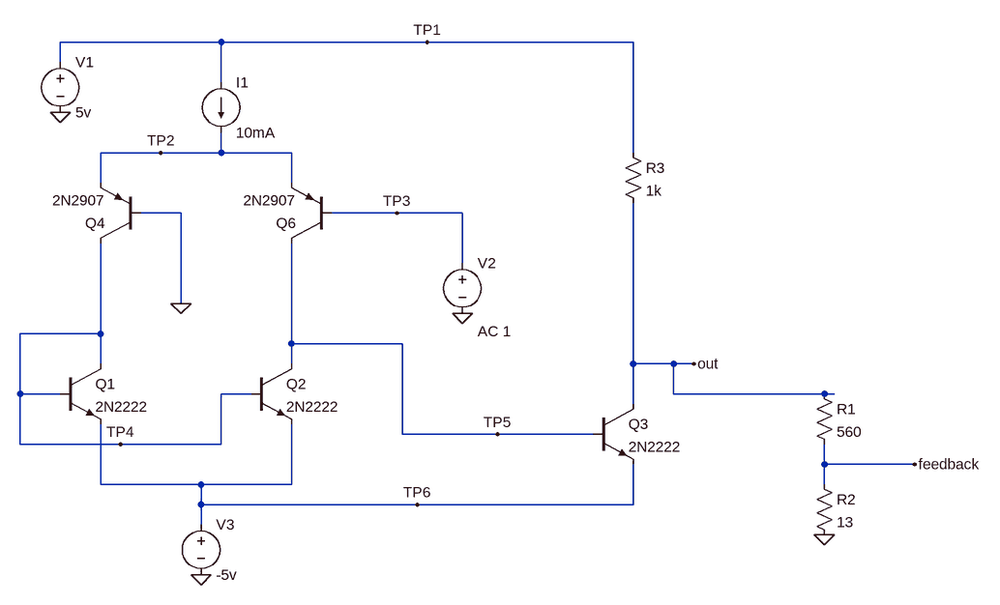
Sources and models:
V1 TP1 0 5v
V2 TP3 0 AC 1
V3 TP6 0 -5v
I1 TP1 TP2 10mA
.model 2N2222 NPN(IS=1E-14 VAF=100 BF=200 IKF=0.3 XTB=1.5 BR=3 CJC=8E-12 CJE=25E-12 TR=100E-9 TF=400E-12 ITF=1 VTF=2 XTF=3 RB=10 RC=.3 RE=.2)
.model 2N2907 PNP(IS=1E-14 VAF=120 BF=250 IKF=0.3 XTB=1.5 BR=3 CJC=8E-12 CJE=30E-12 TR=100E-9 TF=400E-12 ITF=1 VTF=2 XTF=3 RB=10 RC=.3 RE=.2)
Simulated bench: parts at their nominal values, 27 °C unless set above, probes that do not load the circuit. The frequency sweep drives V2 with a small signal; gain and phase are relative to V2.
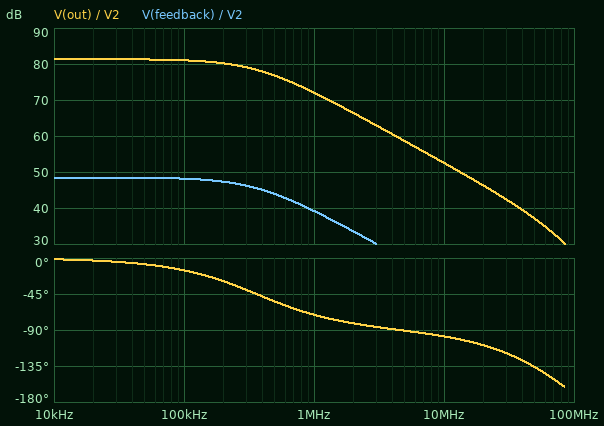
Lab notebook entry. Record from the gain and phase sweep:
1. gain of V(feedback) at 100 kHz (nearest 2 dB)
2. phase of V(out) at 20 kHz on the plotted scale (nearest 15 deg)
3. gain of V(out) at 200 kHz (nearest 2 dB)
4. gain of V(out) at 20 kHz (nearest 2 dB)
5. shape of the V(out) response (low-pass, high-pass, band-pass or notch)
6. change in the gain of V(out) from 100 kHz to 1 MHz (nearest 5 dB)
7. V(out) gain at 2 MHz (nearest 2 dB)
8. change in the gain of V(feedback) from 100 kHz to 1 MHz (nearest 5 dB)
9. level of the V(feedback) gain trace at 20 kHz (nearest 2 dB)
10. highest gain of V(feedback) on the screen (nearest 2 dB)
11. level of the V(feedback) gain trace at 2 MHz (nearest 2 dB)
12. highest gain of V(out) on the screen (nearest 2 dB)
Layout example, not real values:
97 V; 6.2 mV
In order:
48 dB; 0 deg; 80 dB; 82 dB; low-pass; -10 dB; 66 dB; -10 dB; 48 dB; 48 dB; 34 dB; 82 dB
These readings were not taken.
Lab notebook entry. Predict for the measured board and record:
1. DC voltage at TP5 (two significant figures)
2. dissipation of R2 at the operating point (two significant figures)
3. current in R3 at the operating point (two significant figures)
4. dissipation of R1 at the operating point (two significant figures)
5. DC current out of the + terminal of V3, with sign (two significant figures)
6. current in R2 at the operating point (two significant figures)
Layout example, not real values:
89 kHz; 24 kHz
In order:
-4.3 V; 110 µW; 6.7 mA; 4.9 mW; -20 mA; 3.0 mA
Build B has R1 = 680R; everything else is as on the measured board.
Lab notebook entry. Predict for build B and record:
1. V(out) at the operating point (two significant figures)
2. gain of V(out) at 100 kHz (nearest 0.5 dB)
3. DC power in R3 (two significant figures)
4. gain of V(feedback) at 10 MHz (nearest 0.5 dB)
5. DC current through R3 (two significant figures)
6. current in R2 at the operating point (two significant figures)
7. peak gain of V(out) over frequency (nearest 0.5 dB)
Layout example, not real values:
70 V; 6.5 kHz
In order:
-1.9 V; 82.0 dB; 48 mW; 18.0 dB; 6.9 mA; 2.7 mA; 82.5 dB
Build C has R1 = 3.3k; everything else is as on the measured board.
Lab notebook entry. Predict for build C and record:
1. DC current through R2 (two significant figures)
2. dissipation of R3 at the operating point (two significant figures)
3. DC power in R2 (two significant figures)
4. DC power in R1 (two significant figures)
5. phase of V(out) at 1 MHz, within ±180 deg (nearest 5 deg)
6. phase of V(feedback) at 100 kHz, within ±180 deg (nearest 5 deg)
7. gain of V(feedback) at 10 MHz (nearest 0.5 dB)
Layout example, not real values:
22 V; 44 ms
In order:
1.0 mA; 71 mW; 14 µW; 3.6 mW; -80 deg; -30 deg; 4.0 dB
